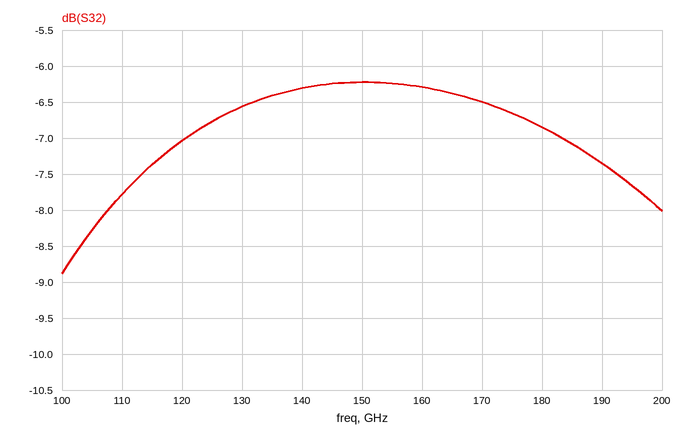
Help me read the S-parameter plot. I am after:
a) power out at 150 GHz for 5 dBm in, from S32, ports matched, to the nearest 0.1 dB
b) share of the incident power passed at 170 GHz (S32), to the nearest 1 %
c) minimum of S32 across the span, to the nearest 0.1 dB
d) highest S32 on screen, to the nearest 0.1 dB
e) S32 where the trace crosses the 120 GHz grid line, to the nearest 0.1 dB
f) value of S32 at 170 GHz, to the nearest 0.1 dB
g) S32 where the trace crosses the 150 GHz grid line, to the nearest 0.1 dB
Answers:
-1.2 dBm
22 %
-8.9 dB
-6.2 dB
-7.0 dB
-6.5 dB
-6.2 dB
